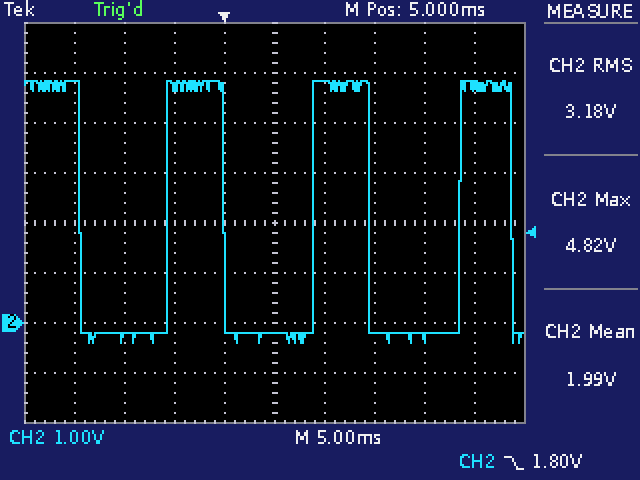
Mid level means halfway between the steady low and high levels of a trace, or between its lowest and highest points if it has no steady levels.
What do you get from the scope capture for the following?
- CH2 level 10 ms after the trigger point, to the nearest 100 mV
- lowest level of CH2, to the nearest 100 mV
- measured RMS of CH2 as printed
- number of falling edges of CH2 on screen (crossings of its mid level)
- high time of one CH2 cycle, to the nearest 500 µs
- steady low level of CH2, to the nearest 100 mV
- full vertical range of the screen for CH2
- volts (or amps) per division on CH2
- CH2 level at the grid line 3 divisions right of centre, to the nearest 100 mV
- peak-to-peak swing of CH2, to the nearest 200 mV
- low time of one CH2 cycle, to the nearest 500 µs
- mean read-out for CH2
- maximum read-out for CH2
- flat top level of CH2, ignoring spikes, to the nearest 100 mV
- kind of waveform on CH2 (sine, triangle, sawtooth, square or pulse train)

4.8 V
-400 mV
3.18 V
4
5.5 ms
-200 mV
8 V
1 V
-300 mV
5.2 V
9.0 ms
1.99 V
4.82 V
4.8 V
pulse train
